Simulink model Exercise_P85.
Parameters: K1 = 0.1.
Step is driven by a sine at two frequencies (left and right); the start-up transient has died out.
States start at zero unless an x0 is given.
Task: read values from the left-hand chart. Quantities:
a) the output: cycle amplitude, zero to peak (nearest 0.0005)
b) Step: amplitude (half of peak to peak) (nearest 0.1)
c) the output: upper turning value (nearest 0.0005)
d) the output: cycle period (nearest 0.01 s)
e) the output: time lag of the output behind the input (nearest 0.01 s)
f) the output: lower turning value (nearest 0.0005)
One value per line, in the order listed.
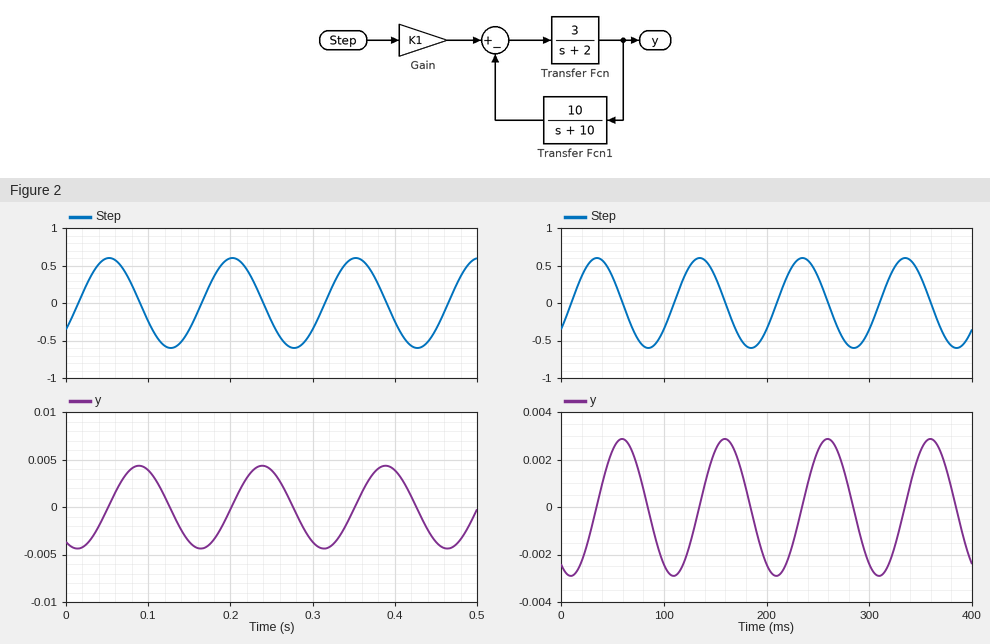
0.0045
0.6
0.0045
0.15 s
0.04 s
-0.0045
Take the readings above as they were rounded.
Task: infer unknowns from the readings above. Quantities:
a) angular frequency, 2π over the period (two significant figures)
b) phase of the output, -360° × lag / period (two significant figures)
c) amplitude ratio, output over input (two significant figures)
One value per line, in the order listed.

42 rad/s
-96°
0.0075
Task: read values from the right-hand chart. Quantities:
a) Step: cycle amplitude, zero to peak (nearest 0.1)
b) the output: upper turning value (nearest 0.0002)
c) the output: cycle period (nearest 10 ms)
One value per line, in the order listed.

0.6
0.0028
100 ms
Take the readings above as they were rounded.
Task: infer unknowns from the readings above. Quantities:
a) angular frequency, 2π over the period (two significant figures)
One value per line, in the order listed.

0.063 rad/ms
